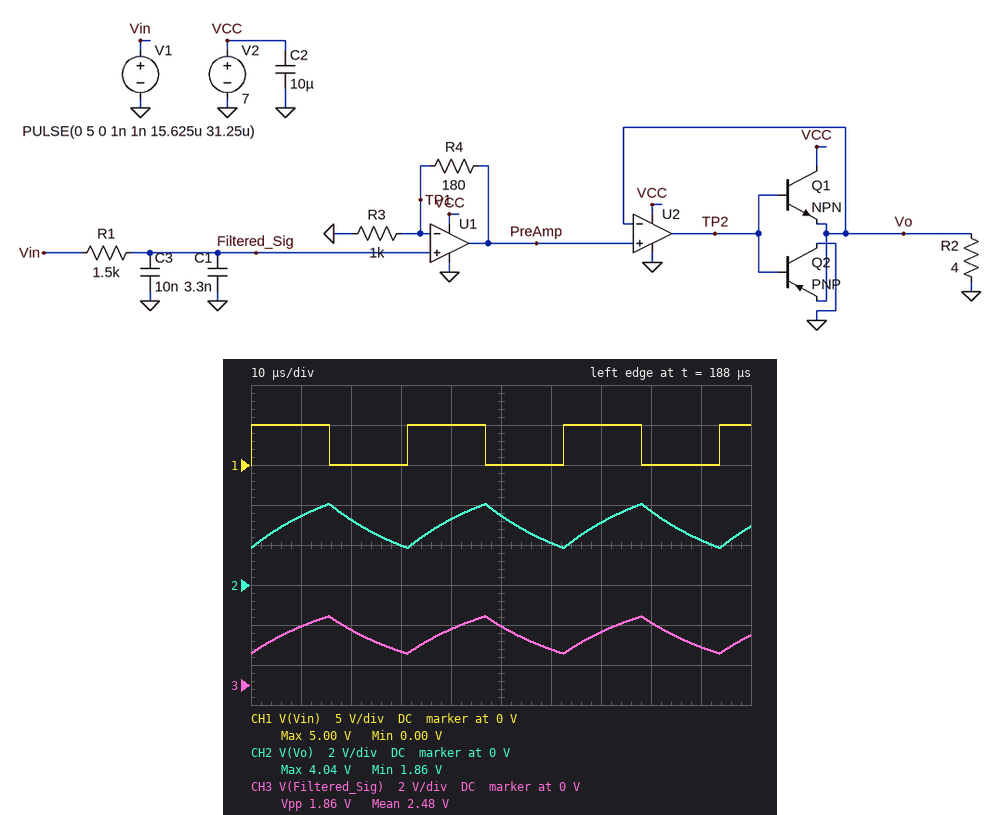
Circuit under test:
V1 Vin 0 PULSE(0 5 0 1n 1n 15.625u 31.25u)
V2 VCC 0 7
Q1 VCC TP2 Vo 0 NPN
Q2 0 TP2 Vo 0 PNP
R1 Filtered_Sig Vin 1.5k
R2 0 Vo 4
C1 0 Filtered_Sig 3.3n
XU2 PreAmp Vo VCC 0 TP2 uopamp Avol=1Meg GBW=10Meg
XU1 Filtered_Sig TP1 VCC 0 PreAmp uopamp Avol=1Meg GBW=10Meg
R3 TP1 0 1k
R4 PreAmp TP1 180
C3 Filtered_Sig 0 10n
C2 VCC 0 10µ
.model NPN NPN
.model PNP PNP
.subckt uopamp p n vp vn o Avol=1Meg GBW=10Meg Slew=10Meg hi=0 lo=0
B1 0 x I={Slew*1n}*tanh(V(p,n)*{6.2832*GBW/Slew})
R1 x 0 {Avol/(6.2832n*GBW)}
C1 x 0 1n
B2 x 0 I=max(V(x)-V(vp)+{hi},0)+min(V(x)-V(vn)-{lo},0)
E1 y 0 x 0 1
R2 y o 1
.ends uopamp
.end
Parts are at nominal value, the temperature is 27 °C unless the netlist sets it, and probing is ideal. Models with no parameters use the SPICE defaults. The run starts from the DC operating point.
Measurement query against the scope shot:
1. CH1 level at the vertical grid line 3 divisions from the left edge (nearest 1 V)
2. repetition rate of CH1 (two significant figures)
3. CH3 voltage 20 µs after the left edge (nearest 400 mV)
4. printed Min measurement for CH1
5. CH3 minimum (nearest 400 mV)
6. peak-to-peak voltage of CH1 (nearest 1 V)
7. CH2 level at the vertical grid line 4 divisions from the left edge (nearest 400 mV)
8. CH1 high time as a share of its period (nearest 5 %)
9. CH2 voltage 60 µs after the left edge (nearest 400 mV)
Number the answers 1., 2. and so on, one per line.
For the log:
1. 0 V
2. 32 kHz
3. 2.8 V
4. 0.00 V
5. 1.6 V
6. 5 V
7. 3.2 V
8. 50 %
9. 2.0 V
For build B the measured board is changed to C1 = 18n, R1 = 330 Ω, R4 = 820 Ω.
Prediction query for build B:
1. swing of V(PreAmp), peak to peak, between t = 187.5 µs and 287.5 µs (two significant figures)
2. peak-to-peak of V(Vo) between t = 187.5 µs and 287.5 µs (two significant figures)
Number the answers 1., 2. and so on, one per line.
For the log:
1. 5.6 V
2. 4.6 V
